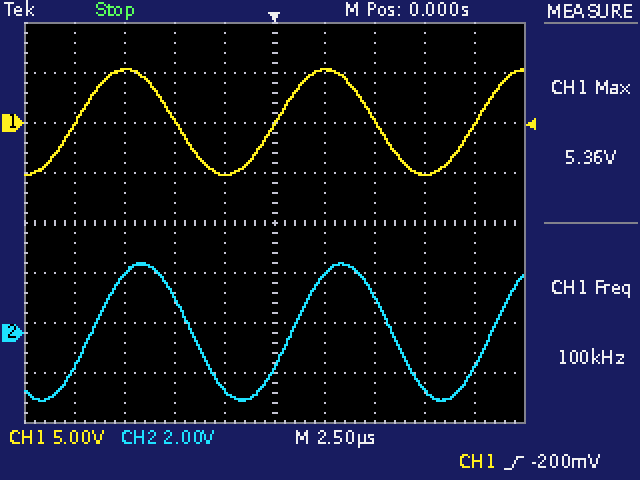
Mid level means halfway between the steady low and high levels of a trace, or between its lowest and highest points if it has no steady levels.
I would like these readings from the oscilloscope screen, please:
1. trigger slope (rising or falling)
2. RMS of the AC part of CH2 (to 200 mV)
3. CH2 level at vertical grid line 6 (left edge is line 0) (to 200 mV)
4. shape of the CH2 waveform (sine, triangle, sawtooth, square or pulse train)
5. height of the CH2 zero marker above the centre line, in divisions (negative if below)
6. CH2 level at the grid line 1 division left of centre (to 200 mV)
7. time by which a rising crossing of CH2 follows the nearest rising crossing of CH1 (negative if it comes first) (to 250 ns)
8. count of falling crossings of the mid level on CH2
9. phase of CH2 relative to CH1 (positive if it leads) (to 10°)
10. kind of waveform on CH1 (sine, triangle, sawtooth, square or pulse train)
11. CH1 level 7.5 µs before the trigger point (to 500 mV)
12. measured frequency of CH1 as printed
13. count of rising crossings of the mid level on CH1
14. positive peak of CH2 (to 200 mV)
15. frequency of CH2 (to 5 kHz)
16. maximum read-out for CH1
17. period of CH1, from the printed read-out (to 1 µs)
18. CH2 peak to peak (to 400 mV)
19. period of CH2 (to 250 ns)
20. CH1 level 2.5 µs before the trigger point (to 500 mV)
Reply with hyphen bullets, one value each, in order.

- rising
- 2.0 V
- 2.4 V
- sine
- -2.2 div
- -2.2 V
- +750 ns
- 2
- -30°
- sine
- 5.5 V
- 100 kHz
- 3
- 2.8 V
- 100 kHz
- 5.36 V
- 10 µs
- 5.6 V
- 10.00 µs
- -5.0 V
